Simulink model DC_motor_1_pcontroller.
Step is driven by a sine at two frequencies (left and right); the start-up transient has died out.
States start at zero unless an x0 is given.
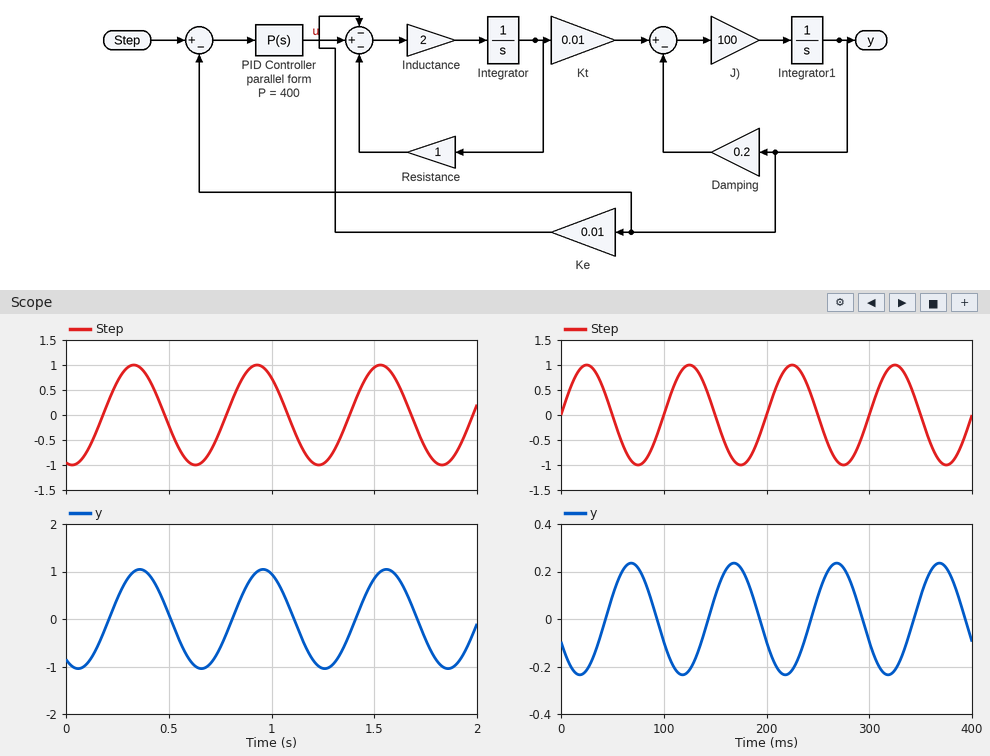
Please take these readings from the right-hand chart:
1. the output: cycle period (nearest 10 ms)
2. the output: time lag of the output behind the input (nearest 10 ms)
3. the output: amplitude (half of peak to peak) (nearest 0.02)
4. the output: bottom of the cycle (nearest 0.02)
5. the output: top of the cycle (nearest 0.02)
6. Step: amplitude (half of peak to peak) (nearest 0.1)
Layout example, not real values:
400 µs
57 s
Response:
100 ms
40 ms
0.24
-0.24
0.24
1.0
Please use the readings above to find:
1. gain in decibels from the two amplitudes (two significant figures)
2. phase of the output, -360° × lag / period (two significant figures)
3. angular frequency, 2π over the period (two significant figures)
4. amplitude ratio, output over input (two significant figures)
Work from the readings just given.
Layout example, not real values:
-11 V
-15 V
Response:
-12 dB
-140°
0.063 rad/ms
0.24
